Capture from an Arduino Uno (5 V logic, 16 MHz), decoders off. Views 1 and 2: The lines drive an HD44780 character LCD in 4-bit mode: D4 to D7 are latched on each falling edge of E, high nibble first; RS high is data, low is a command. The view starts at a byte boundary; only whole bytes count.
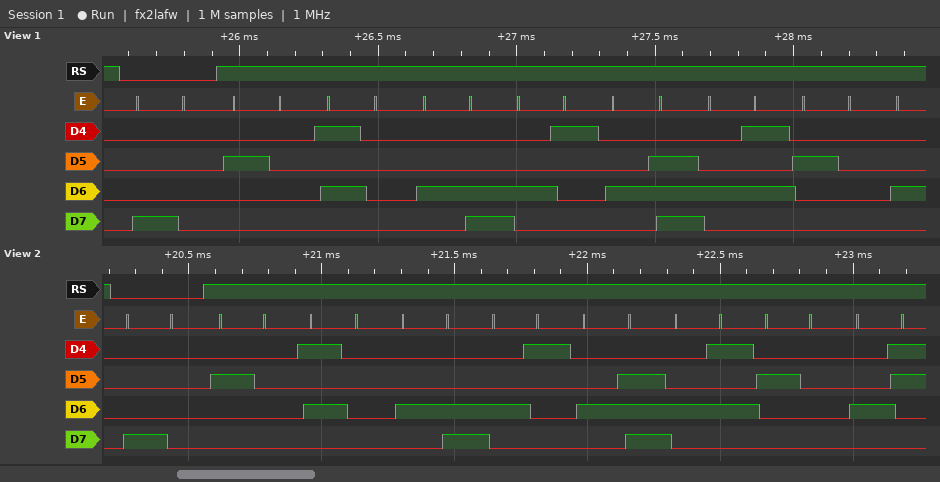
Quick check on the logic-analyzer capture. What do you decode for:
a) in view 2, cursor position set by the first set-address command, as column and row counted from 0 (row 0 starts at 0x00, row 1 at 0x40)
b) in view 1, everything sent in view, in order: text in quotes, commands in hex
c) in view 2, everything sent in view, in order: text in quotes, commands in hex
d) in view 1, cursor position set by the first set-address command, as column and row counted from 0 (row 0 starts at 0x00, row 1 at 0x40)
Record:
column 0, row 0
0x80 " PLANE "
0x80 " PLANE C"
column 0, row 0
